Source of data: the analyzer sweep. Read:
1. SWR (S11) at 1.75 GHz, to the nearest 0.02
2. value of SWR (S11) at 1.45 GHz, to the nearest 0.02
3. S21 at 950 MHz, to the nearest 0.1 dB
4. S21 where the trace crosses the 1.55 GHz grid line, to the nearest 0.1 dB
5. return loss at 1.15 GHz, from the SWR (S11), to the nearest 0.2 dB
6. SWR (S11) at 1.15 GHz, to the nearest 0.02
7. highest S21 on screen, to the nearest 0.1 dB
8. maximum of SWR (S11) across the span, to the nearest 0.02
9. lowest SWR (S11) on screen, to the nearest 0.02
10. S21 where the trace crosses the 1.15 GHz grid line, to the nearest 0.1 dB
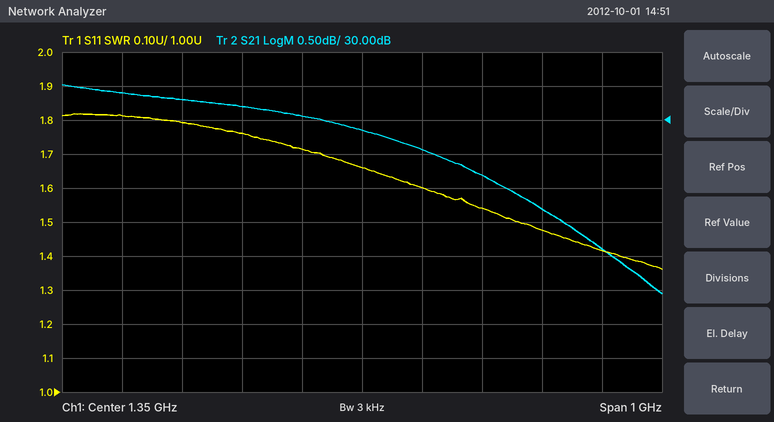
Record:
1.42
1.60
30.4 dB
29.2 dB
11.2 dB
1.76
30.5 dB
1.82
1.36
30.2 dB
